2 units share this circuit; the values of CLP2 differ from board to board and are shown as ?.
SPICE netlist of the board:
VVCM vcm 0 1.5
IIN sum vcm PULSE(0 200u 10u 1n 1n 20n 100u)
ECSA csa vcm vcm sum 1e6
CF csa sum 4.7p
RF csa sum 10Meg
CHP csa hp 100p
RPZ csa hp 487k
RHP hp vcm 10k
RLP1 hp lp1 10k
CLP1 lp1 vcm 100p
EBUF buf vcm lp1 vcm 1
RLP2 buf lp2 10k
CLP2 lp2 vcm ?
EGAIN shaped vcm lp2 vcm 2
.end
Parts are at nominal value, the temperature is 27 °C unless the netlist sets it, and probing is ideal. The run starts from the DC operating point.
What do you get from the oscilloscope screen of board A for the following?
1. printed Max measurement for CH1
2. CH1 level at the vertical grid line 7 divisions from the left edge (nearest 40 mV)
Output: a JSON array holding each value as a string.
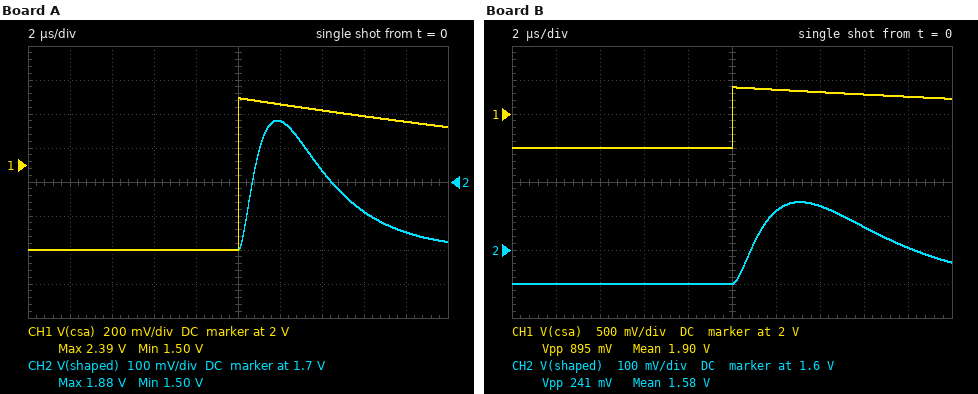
["2.39 V", "2.32 V"]
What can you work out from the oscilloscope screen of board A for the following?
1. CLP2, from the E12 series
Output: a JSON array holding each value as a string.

["82 pF"]
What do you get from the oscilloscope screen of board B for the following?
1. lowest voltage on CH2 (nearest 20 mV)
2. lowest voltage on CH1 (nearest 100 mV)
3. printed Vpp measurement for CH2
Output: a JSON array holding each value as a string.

["1.50 V", "1.5 V", "241 mV"]
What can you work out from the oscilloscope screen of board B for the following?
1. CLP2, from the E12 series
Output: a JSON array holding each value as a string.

["270 pF"]
